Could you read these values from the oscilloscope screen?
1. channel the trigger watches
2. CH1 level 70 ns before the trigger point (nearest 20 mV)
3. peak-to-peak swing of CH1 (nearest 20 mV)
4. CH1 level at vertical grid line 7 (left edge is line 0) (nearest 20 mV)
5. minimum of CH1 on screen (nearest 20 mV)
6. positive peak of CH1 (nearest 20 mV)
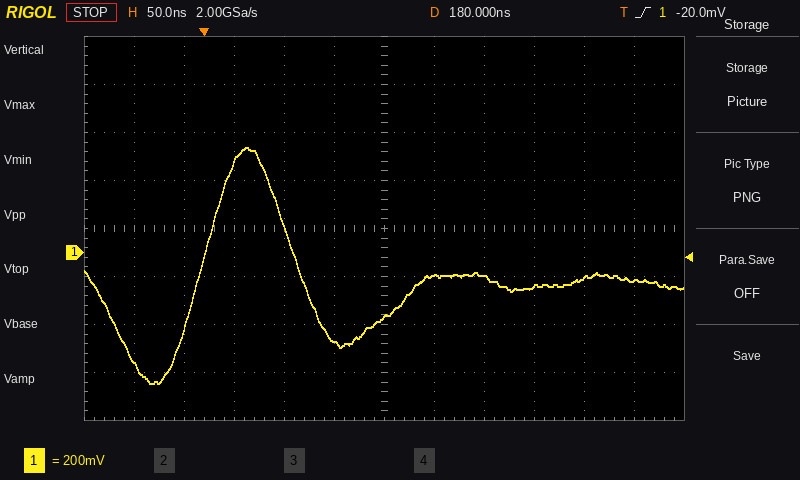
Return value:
CH1
-460 mV
980 mV
-100 mV
-540 mV
440 mV
